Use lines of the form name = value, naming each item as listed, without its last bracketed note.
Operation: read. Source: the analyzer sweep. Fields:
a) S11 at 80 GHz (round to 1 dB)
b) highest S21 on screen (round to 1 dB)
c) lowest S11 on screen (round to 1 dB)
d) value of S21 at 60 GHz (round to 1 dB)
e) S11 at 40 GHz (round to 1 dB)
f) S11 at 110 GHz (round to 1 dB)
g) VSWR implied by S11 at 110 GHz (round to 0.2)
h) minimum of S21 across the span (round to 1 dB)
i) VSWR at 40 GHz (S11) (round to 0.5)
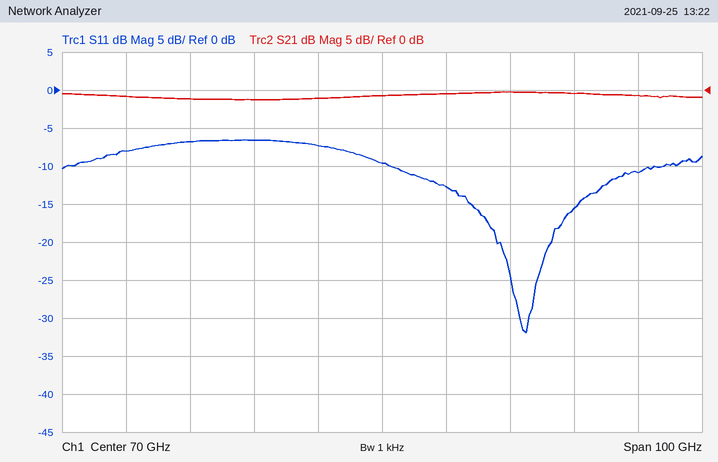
S11 at 80 GHz = -13 dB
highest S21 on screen = 0 dB
lowest S11 on screen = -32 dB
value of S21 at 60 GHz = -1 dB
S11 at 40 GHz = -7 dB
S11 at 110 GHz = -11 dB
VSWR implied by S11 at 110 GHz = 1.8
minimum of S21 across the span = -1 dB
VSWR at 40 GHz (S11) = 2.5
